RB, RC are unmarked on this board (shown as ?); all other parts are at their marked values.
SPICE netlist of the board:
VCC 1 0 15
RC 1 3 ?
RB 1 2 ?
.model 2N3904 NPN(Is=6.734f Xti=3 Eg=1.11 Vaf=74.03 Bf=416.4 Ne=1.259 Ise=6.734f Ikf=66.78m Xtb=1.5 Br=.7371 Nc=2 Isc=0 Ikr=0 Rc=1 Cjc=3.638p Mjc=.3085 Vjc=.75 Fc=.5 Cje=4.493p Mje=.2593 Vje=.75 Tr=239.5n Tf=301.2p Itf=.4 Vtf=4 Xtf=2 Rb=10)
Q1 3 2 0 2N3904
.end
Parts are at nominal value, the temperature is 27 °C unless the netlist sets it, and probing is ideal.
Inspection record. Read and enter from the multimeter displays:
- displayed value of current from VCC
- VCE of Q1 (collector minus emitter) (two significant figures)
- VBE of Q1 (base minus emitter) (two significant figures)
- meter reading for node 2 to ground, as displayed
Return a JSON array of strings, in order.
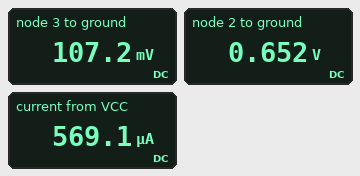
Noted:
["569.1 µA", "110 mV", "650 mV", "0.652 V"]
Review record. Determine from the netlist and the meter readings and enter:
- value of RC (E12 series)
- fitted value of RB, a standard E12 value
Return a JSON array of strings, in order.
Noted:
["27 kΩ", "820 kΩ"]
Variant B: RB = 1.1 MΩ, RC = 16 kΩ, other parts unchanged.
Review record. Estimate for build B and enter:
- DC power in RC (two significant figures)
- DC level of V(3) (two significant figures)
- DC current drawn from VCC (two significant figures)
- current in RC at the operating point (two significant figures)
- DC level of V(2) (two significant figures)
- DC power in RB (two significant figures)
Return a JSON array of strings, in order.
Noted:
["14 mW", "140 mV", "940 µA", "930 µA", "660 mV", "190 µW"]
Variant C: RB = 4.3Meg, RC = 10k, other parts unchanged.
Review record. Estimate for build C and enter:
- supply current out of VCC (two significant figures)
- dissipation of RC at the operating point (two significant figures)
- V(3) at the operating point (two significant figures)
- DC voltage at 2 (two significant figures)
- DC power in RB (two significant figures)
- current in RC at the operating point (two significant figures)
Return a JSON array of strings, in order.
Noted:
["450 µA", "2.0 mW", "11 V", "640 mV", "48 µW", "440 µA"]
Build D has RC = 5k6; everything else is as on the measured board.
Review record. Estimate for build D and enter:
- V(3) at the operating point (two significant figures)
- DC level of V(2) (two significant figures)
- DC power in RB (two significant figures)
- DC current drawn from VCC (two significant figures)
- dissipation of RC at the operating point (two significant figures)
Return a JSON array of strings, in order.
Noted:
["570 mV", "690 mV", "250 µW", "2.6 mA", "37 mW"]
